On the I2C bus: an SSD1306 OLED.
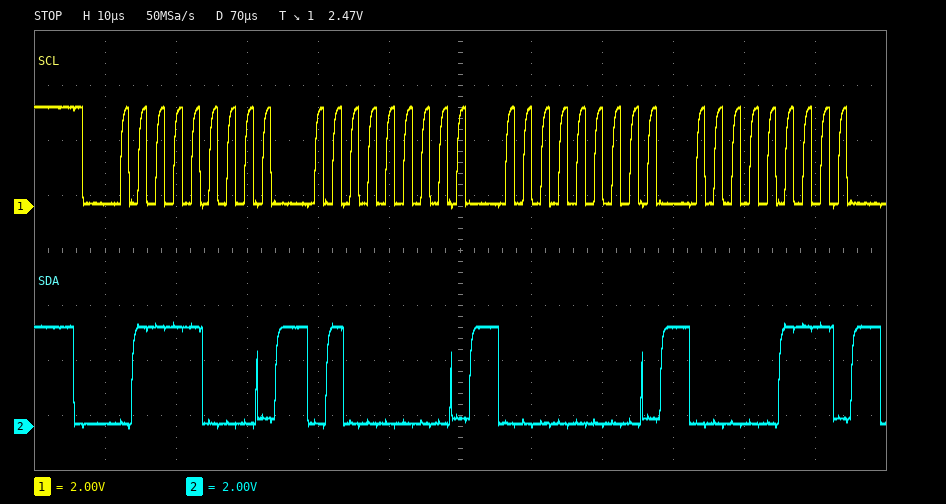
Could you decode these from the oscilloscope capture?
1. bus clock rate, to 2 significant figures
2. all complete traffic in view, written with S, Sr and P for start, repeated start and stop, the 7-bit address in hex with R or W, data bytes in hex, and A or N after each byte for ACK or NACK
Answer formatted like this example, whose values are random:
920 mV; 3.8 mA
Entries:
400 kHz; S 3CW A 40 A 00 A 07 A
